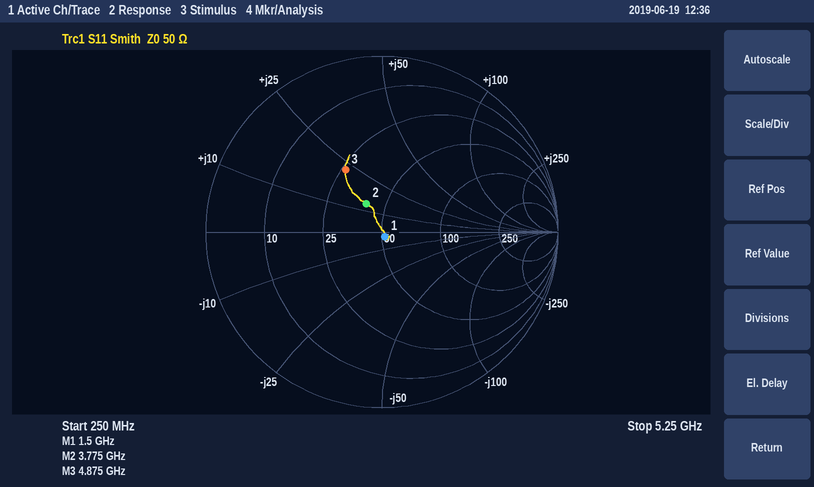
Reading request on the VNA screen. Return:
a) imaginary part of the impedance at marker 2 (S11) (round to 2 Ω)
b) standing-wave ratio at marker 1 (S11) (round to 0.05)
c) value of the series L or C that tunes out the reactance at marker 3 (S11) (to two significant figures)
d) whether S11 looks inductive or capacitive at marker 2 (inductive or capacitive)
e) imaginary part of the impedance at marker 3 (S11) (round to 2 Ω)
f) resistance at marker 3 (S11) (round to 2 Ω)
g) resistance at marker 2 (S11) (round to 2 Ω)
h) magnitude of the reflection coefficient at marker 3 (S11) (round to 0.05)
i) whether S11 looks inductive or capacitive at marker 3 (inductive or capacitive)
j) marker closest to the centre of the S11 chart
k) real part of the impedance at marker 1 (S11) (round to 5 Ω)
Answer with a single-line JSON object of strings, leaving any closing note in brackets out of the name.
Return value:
{"imaginary part of the impedance at marker 2 (S11)": "+14 Ω", "standing-wave ratio at marker 1 (S11)": "1.05", "value of the series L or C that tunes out the reactance at marker 3 (S11)": "1.5 pF", "whether S11 looks inductive or capacitive at marker 2": "inductive", "imaginary part of the impedance at marker 3 (S11)": "+22 Ω", "resistance at marker 3 (S11)": "26 Ω", "resistance at marker 2 (S11)": "40 Ω", "magnitude of the reflection coefficient at marker 3 (S11)": "0.40", "whether S11 looks inductive or capacitive at marker 3": "inductive", "marker closest to the centre of the S11 chart": "marker 1", "real part of the impedance at marker 1 (S11)": "50 Ω"}
